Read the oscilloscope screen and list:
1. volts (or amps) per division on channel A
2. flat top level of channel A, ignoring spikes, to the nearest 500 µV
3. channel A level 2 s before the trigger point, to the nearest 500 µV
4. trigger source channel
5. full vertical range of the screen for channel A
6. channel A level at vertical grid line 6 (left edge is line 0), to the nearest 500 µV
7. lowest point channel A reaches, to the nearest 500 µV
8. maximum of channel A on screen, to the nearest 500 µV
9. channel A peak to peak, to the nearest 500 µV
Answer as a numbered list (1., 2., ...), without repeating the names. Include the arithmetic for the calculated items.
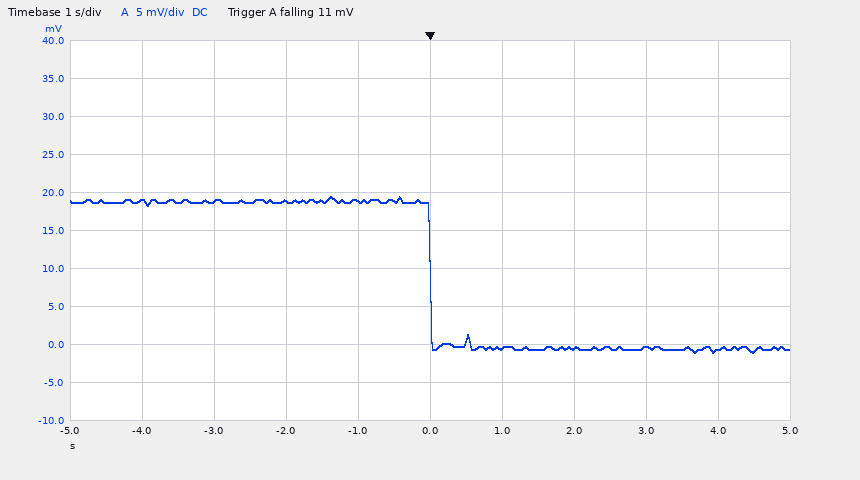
1. 5 mV
2. 18.5 mV
3. 19.0 mV
4. channel A
5. 50 mV
6. -500 µV
7. -1.0 mV
8. 19.5 mV
9. 19.5 mV − (-1.0 mV) = 20.5 mV
